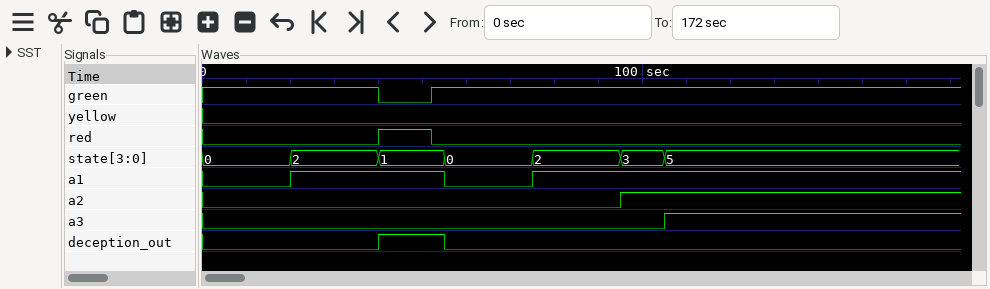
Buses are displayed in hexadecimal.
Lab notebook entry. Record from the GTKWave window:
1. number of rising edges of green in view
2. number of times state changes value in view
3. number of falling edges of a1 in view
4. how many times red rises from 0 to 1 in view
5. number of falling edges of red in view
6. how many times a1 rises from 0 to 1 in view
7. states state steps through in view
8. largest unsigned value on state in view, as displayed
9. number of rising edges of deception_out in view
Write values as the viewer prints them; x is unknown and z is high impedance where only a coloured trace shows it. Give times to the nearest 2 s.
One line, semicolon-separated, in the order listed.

1; 6; 1; 1; 1; 2; 0, 2, 1, 0, 2, 3, 5; 5; 1
